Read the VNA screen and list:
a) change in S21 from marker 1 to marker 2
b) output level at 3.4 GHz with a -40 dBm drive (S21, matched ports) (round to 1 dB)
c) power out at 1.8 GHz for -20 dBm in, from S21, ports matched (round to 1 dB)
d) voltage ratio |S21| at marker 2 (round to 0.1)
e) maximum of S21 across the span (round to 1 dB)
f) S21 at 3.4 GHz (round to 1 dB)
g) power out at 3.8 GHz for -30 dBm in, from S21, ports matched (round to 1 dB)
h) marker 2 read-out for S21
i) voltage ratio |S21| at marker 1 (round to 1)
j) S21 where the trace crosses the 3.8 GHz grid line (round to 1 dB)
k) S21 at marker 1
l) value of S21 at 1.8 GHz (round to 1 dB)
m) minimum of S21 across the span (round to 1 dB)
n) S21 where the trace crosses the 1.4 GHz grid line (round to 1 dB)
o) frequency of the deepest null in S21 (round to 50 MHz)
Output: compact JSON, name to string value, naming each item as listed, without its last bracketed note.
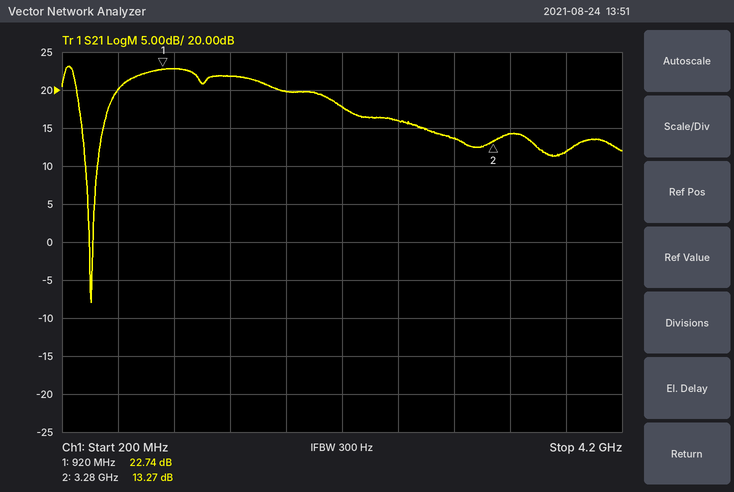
{"change in S21 from marker 1 to marker 2": "-9.47 dB", "output level at 3.4 GHz with a -40 dBm drive (S21, matched ports)": "-26 dBm", "power out at 1.8 GHz for -20 dBm in, from S21, ports matched": "0 dBm", "voltage ratio |S21| at marker 2": "4.6", "maximum of S21 across the span": "23 dB", "S21 at 3.4 GHz": "14 dB", "power out at 3.8 GHz for -30 dBm in, from S21, ports matched": "-18 dBm", "marker 2 read-out for S21": "13.27 dB", "voltage ratio |S21| at marker 1": "14", "S21 where the trace crosses the 3.8 GHz grid line": "12 dB", "S21 at marker 1": "22.74 dB", "value of S21 at 1.8 GHz": "20 dB", "minimum of S21 across the span": "-8 dB", "S21 where the trace crosses the 1.4 GHz grid line": "22 dB", "frequency of the deepest null in S21": "400 MHz"}
